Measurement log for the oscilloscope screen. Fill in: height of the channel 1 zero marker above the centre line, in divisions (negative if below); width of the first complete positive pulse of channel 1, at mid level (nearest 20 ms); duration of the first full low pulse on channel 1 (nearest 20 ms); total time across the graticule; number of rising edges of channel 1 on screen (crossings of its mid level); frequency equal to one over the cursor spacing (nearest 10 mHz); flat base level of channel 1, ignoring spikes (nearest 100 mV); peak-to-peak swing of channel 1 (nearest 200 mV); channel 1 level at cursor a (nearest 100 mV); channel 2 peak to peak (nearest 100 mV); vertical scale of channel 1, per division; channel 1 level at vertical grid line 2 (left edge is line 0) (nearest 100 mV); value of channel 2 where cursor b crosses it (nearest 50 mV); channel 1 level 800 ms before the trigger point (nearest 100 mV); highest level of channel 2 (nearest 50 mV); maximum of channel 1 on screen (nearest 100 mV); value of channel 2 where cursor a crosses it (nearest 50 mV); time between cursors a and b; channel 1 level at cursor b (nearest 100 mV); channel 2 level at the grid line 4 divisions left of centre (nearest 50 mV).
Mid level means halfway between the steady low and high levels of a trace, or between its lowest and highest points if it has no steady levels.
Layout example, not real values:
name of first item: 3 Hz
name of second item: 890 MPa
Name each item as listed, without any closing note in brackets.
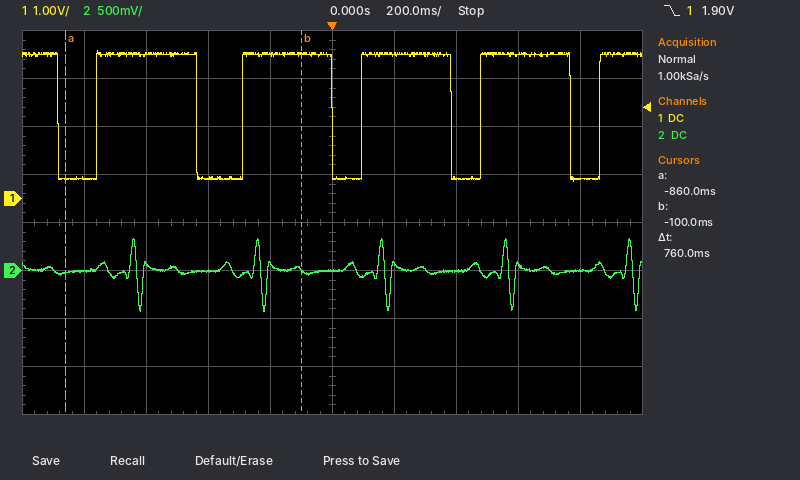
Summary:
height of the channel 1 zero marker above the centre line, in divisions: +0.5 div
width of the first complete positive pulse of channel 1, at mid level: 320 ms
duration of the first full low pulse on channel 1: 120 ms
total time across the graticule: 2 s
number of rising edges of channel 1 on screen: 5
frequency equal to one over the cursor spacing: 1.32 Hz
flat base level of channel 1, ignoring spikes: 400 mV
peak-to-peak swing of channel 1: 2.8 V
channel 1 level at cursor a: 400 mV
channel 2 peak to peak: 800 mV
vertical scale of channel 1, per division: 1 V
channel 1 level at vertical grid line 2 (left edge is line 0): 3.0 V
value of channel 2 where cursor b crosses it: 0 mV
channel 1 level 800 ms before the trigger point: 400 mV
highest level of channel 2: 350 mV
maximum of channel 1 on screen: 3.1 V
value of channel 2 where cursor a crosses it: 0 mV
time between cursors a and b: 760 ms
channel 1 level at cursor b: 3.0 V
channel 2 level at the grid line 4 divisions left of centre: 0 mV
